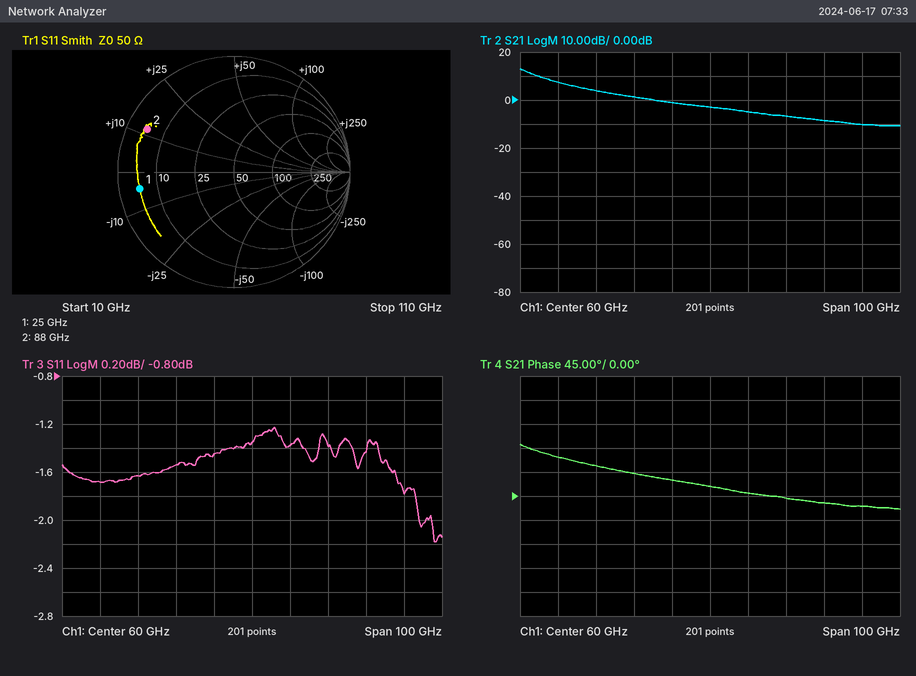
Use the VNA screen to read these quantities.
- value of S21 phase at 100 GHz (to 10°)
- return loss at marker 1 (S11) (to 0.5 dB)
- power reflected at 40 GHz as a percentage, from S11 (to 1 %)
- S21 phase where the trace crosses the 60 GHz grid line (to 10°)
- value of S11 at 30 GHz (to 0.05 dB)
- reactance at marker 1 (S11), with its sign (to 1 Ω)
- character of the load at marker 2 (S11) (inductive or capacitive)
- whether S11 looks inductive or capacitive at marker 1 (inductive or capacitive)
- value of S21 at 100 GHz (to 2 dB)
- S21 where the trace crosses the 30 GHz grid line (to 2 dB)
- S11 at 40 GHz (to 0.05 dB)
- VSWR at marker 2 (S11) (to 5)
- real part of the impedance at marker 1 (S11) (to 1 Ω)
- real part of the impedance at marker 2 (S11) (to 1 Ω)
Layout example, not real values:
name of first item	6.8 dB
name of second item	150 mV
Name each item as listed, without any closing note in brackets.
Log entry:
value of S21 phase at 100 GHz	-20°
return loss at marker 1 (S11)	1.5 dB
power reflected at 40 GHz as a percentage, from S11	70 %
S21 phase where the trace crosses the 60 GHz grid line	20°
value of S11 at 30 GHz	-1.65 dB
reactance at marker 1 (S11), with its sign	-4 Ω
character of the load at marker 2 (S11)	inductive
whether S11 looks inductive or capacitive at marker 1	capacitive
value of S21 at 100 GHz	-10 dB
S21 where the trace crosses the 30 GHz grid line	4 dB
S11 at 40 GHz	-1.55 dB
VSWR at marker 2 (S11)	10
real part of the impedance at marker 1 (S11)	5 Ω
real part of the impedance at marker 2 (S11)	5 Ω
